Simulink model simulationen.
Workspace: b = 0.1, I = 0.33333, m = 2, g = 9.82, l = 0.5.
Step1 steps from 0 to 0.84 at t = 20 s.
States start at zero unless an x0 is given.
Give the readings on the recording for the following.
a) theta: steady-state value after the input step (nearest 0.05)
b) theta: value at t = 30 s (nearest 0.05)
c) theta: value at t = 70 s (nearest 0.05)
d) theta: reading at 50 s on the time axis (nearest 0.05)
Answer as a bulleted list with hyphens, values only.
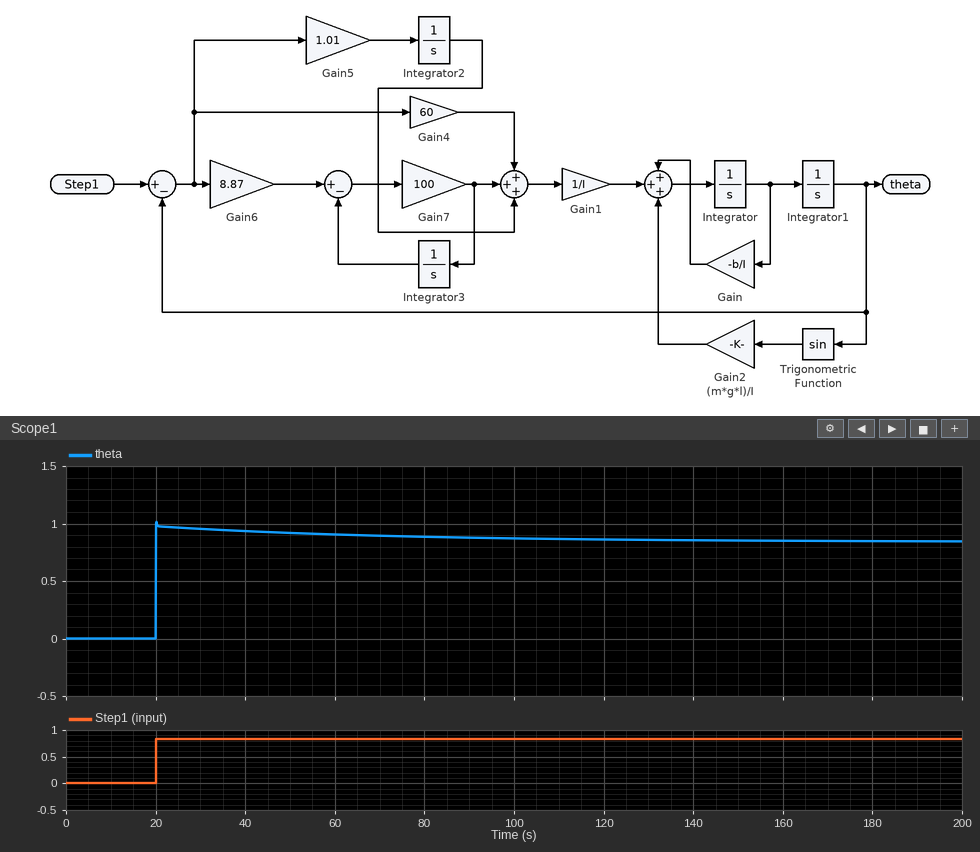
- 0.85
- 0.95
- 0.90
- 0.90
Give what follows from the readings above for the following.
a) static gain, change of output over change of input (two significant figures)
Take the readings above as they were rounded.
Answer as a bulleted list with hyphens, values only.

- 1.0
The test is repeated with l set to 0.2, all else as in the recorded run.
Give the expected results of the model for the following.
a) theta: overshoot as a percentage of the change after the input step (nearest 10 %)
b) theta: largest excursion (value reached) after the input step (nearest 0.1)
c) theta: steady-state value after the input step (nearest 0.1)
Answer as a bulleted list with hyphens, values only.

- 20 %
- 1.0
- 0.8
